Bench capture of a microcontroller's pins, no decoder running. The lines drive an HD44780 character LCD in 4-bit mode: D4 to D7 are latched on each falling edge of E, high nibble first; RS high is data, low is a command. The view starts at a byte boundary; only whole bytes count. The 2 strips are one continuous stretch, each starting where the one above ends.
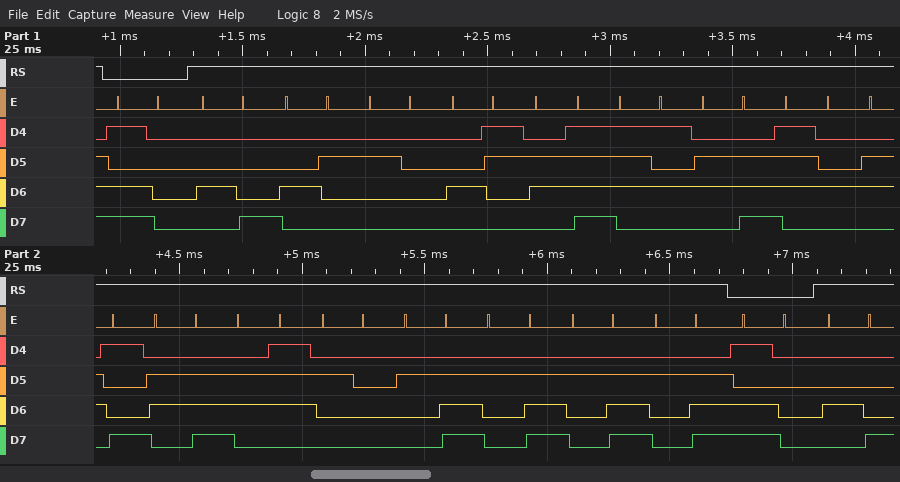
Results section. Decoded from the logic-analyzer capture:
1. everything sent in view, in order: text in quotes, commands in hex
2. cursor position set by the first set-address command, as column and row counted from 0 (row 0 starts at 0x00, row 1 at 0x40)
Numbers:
0xD0 "HB Counting ...." 0xD0 "H"
column 16, row 1
